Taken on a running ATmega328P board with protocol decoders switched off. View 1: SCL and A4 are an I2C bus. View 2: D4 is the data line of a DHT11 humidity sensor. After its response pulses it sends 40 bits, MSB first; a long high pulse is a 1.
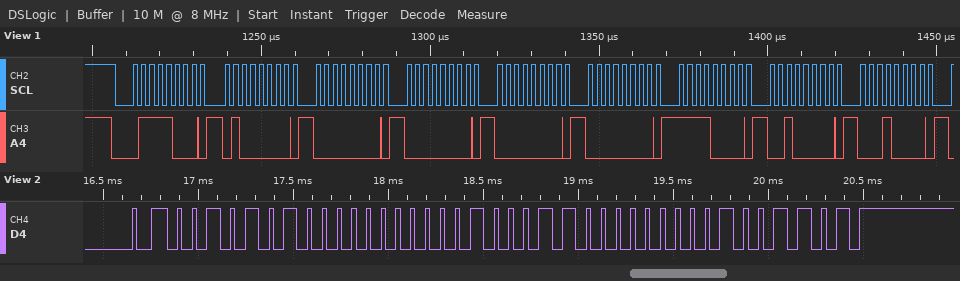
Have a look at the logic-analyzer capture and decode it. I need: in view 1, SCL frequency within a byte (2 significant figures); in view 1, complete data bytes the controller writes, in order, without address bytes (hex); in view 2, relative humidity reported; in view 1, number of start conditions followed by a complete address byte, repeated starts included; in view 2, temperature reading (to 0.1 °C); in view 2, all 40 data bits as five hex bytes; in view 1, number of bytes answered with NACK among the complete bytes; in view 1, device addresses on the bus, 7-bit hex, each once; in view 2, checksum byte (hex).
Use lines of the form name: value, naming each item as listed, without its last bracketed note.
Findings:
in view 1, SCL frequency within a byte: 400 kHz
in view 1, complete data bytes the controller writes, in order, without address bytes: 40 00 00 00 00 F0 20 10
in view 2, relative humidity reported: 42 %
in view 1, number of start conditions followed by a complete address byte, repeated starts included: 1
in view 2, temperature reading: 35.0 °C
in view 2, all 40 data bits as five hex bytes: 2A 00 23 00 4D
in view 1, number of bytes answered with NACK among the complete bytes: 0
in view 1, device addresses on the bus, 7-bit hex, each once: 0x3C
in view 2, checksum byte: 0x4D
